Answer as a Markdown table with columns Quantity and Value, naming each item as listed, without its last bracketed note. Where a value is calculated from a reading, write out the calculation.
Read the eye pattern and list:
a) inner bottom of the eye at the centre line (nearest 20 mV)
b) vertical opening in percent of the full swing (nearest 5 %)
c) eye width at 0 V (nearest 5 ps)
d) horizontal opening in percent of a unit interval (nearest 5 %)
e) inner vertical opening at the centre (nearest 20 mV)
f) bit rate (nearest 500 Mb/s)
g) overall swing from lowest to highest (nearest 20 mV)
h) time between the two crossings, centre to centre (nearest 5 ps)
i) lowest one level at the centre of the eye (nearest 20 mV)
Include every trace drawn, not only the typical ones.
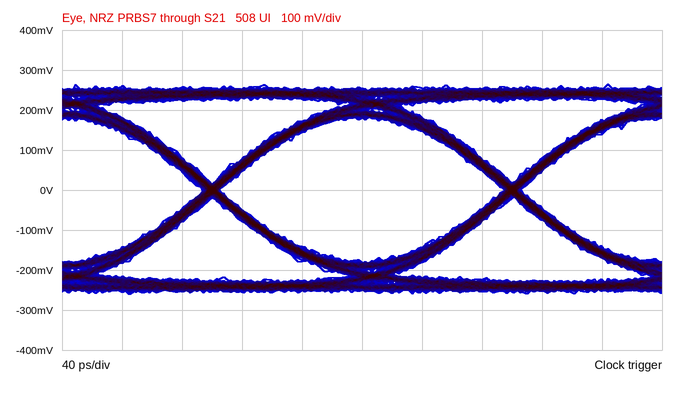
| Quantity | Value |
|---|---|
| inner bottom of the eye at the centre line | -180 mV |
| vertical opening in percent of the full swing | 360 mV / 520 mV ≈ 69.2 %, so 70 % to the nearest 5 % |
| eye width at 0 V | 190 ps |
| horizontal opening in percent of a unit interval | 190 ps / 200 ps ≈ 95 % |
| inner vertical opening at the centre | 360 mV |
| bit rate | 5.0 Gb/s |
| overall swing from lowest to highest | 520 mV |
| time between the two crossings, centre to centre | 200 ps |
| lowest one level at the centre of the eye | 180 mV |
